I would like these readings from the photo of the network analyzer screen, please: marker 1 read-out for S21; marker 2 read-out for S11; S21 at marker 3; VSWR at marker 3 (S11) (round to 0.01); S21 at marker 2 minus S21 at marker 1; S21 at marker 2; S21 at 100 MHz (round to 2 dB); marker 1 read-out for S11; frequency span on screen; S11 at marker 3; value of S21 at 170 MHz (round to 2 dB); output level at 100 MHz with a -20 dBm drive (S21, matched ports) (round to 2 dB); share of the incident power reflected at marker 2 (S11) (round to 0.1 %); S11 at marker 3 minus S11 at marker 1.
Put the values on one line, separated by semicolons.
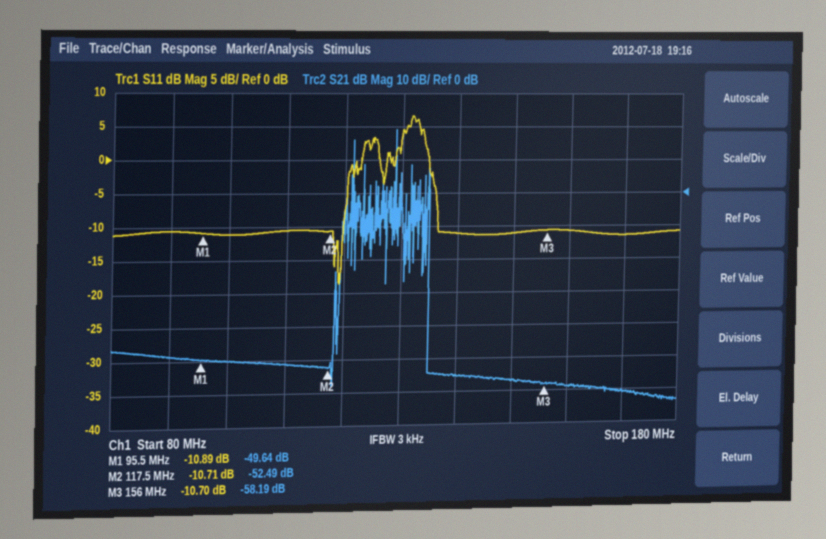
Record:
-49.64 dB; -10.71 dB; -58.19 dB; 1.82; -2.85 dB; -52.49 dB; -50 dB; -10.89 dB; 100 MHz; -10.70 dB; -60 dB; -70 dBm; 8.5 %; 0.19 dB
